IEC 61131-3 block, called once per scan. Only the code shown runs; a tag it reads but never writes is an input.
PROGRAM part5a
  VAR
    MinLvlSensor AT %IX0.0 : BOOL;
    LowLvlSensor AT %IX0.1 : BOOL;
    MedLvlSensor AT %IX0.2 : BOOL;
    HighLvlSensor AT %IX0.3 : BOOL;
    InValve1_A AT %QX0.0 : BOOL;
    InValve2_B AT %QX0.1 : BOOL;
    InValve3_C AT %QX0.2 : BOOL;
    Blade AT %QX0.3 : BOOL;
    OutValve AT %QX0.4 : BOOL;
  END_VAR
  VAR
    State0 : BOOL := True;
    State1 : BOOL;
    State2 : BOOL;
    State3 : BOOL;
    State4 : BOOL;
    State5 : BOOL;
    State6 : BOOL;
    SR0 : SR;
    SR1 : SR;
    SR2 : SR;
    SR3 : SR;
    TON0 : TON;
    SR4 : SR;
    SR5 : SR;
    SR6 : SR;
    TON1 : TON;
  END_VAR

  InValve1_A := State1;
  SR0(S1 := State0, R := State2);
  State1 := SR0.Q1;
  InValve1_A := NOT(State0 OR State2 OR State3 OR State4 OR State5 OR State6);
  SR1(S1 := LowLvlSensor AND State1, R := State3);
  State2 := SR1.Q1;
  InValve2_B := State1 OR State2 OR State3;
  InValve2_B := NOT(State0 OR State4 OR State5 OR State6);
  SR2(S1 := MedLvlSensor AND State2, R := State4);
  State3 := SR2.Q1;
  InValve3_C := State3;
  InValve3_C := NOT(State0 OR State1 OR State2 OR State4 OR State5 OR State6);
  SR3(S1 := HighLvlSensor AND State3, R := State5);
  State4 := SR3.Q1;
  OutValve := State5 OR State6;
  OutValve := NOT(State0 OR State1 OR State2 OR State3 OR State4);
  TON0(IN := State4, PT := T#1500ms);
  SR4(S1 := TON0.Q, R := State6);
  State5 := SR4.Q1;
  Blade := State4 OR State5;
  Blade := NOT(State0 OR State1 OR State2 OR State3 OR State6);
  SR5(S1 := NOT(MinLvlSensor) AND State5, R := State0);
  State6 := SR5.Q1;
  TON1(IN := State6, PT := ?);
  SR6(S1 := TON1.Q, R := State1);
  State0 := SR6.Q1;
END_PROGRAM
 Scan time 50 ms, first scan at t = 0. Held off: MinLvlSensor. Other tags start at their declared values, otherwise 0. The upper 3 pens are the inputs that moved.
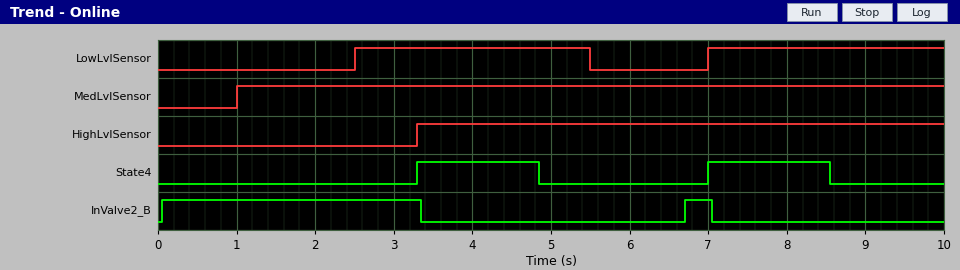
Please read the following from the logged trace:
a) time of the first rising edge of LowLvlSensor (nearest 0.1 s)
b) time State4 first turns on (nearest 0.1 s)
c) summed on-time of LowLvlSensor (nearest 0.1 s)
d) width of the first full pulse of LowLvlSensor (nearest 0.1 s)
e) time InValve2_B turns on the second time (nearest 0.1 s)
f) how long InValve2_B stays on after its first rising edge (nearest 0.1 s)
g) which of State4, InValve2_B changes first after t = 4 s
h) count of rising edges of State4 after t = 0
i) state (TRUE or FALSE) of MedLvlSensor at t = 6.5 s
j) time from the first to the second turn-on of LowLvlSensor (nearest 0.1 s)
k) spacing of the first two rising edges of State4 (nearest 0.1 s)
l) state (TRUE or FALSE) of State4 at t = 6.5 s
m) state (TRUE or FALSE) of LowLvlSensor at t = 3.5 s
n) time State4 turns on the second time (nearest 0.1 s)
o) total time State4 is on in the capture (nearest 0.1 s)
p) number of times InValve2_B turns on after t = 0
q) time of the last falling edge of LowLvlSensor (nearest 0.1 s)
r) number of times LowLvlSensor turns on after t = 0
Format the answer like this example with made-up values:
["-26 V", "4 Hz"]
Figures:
["2.5 s", "3.3 s", "6.0 s", "3.0 s", "6.7 s", "3.3 s", "State4", "2", "TRUE", "4.5 s", "3.7 s", "FALSE", "TRUE", "7.0 s", "3.1 s", "2", "5.5 s", "2"]
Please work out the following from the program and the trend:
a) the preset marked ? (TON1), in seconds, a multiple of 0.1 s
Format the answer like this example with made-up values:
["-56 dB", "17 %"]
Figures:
["1.8 s"]
